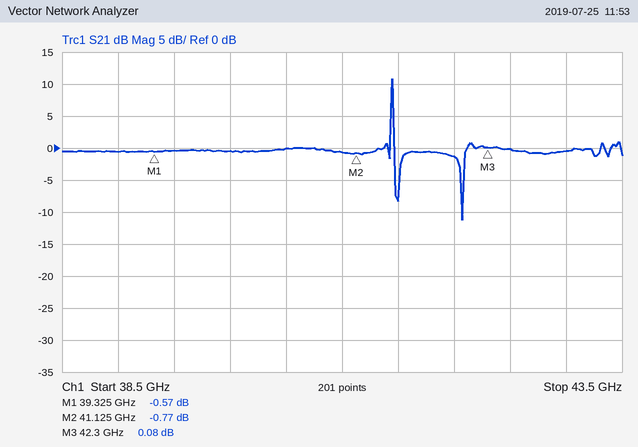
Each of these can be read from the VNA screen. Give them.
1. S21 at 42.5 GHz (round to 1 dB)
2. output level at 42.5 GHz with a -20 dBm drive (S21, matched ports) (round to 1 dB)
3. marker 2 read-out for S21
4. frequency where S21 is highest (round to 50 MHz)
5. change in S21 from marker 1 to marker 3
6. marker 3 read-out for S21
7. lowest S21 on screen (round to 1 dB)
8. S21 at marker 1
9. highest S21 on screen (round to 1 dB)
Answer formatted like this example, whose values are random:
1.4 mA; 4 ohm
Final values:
0 dB; -20 dBm; -0.77 dB; 41.45 GHz; 0.65 dB; 0.08 dB; -11 dB; -0.57 dB; 11 dB
